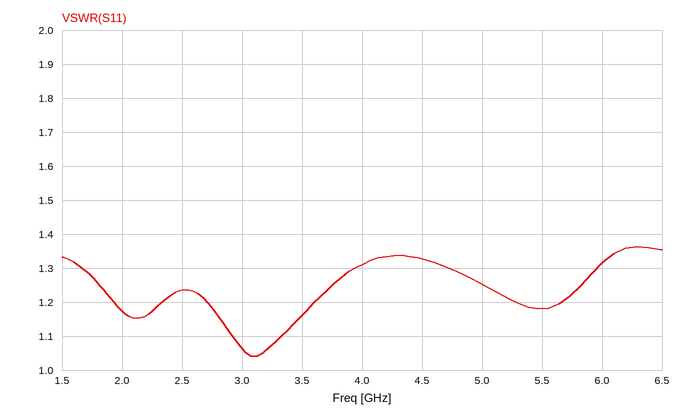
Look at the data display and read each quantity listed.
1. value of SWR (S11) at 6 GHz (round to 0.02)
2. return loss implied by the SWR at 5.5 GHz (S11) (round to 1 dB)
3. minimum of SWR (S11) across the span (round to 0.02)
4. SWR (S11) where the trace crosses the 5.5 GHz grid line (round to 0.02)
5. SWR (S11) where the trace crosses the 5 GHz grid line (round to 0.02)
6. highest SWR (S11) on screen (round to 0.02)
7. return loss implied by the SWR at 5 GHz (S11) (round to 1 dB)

1.32
22 dB
1.04
1.18
1.26
1.36
19 dB
